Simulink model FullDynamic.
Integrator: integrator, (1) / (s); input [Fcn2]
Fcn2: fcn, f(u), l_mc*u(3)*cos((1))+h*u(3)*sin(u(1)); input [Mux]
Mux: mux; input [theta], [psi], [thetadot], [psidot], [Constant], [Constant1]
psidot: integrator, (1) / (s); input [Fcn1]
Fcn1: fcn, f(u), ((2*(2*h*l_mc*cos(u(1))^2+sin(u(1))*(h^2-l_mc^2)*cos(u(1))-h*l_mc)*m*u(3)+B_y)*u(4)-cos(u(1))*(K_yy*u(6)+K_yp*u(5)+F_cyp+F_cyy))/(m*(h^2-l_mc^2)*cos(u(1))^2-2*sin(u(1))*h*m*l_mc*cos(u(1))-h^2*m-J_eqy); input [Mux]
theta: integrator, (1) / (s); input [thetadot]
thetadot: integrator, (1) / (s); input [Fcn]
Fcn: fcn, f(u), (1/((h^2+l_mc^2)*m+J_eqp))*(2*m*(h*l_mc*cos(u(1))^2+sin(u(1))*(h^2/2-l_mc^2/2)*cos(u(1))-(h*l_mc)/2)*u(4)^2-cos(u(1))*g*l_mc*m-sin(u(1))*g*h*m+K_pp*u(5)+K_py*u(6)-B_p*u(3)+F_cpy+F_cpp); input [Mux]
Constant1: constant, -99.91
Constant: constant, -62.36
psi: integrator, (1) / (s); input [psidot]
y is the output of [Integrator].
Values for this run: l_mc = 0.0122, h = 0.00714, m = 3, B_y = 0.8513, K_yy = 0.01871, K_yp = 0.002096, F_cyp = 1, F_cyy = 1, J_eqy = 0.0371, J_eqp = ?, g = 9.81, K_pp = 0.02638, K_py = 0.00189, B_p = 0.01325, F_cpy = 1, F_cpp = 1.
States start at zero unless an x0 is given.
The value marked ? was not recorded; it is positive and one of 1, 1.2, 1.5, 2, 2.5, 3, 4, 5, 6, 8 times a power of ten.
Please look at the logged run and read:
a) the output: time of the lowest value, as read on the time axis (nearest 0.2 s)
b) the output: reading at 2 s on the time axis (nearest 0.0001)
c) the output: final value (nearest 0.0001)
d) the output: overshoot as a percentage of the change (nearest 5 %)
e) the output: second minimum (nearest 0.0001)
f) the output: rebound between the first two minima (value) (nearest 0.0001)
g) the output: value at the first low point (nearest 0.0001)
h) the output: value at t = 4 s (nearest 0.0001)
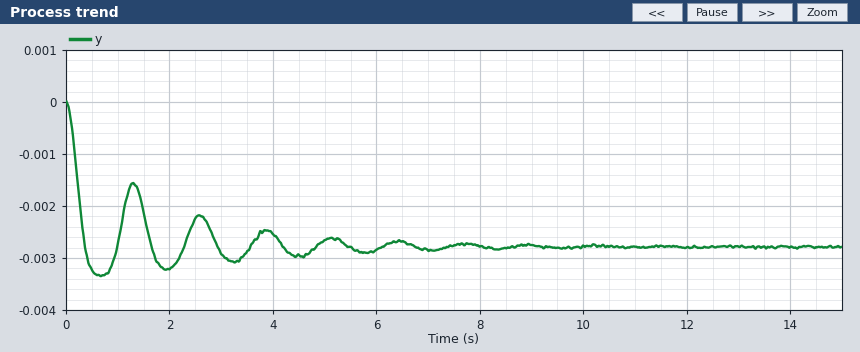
0.6 s
-0.0032
-0.0028
20 %
-0.0032
-0.0016
-0.0033
-0.0025
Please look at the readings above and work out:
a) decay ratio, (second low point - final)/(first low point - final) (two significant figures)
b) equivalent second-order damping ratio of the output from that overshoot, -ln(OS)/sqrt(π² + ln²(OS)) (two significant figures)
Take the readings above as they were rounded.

0.80
0.46
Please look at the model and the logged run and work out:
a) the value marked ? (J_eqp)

0.015
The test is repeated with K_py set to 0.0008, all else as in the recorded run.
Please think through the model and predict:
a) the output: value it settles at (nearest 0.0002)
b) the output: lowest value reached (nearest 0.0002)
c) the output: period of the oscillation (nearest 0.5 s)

-0.0018
-0.0026
1.5 s
